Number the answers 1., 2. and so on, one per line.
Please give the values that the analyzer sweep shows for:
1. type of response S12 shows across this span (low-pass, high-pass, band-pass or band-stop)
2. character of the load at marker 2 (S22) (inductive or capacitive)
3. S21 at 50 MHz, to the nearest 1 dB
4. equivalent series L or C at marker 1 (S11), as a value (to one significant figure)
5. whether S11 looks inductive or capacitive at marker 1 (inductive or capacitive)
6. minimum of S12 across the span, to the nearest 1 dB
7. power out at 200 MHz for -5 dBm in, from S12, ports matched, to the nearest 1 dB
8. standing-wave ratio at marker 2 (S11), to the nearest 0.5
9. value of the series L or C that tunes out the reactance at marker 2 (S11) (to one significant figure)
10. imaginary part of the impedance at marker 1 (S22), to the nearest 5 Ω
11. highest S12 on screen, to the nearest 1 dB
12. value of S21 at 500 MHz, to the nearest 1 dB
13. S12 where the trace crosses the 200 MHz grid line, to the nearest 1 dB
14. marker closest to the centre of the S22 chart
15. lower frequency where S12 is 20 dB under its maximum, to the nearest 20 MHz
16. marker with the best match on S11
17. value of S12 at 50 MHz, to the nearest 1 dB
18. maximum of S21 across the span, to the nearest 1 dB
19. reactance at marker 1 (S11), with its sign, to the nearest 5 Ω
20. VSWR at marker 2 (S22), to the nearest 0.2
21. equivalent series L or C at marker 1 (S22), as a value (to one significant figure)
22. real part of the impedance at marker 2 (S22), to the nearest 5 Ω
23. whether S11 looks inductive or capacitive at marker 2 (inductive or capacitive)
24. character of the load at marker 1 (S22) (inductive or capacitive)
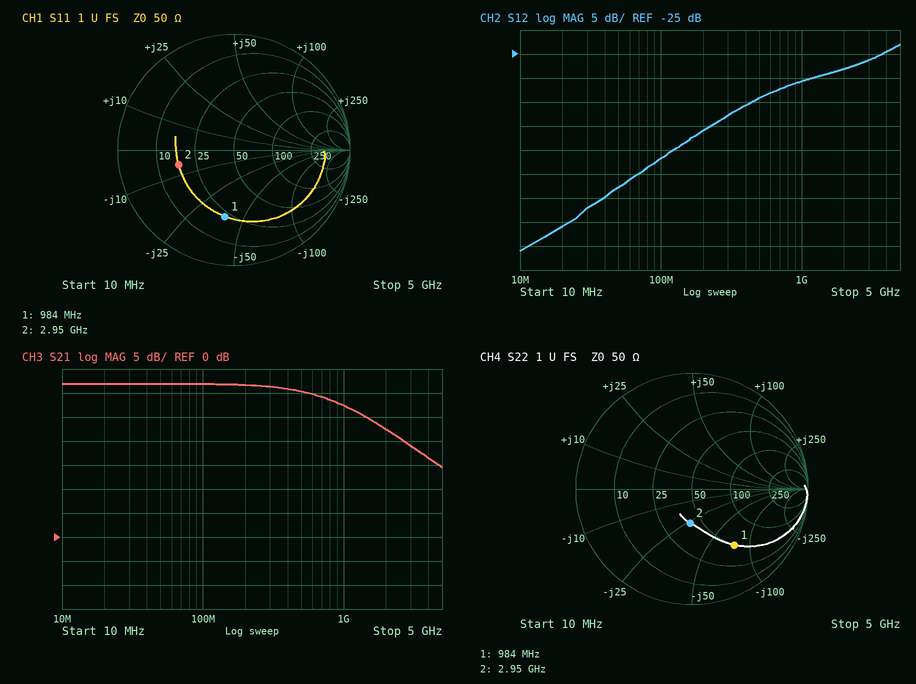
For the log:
1. high-pass
2. capacitive
3. 32 dB
4. 4 pF
5. capacitive
6. -66 dB
7. -46 dBm
8. 3.0
9. 300 pH
10. -75 Ω
11. -23 dB
12. 30 dB
13. -41 dB
14. marker 2
15. 160 MHz
16. marker 2
17. -53 dB
18. 32 dB
19. -40 Ω
20. 1.8
21. 2 pF
22. 40 Ω
23. capacitive
24. capacitive
